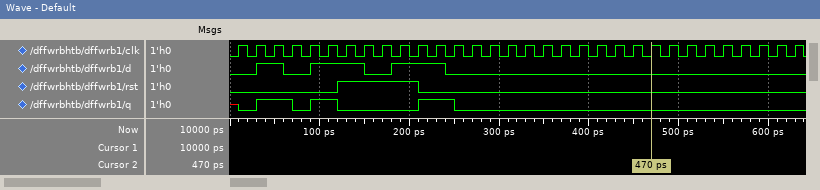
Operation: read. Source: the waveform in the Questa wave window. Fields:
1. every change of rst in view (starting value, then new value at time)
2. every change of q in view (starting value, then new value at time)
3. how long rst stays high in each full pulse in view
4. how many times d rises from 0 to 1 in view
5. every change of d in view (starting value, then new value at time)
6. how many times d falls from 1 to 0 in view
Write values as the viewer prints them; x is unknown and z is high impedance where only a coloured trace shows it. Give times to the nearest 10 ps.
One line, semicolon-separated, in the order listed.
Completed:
0, 1 at 120 ps, 0 at 210 ps; x, 0 at 10 ps, 1 at 30 ps, 0 at 70 ps, 1 at 90 ps, 0 at 120 ps, 1 at 210 ps, 0 at 250 ps; 90 ps; 3; 0, 1 at 30 ps, 0 at 60 ps, 1 at 90 ps, 0 at 150 ps, 1 at 180 ps, 0 at 240 ps; 3
